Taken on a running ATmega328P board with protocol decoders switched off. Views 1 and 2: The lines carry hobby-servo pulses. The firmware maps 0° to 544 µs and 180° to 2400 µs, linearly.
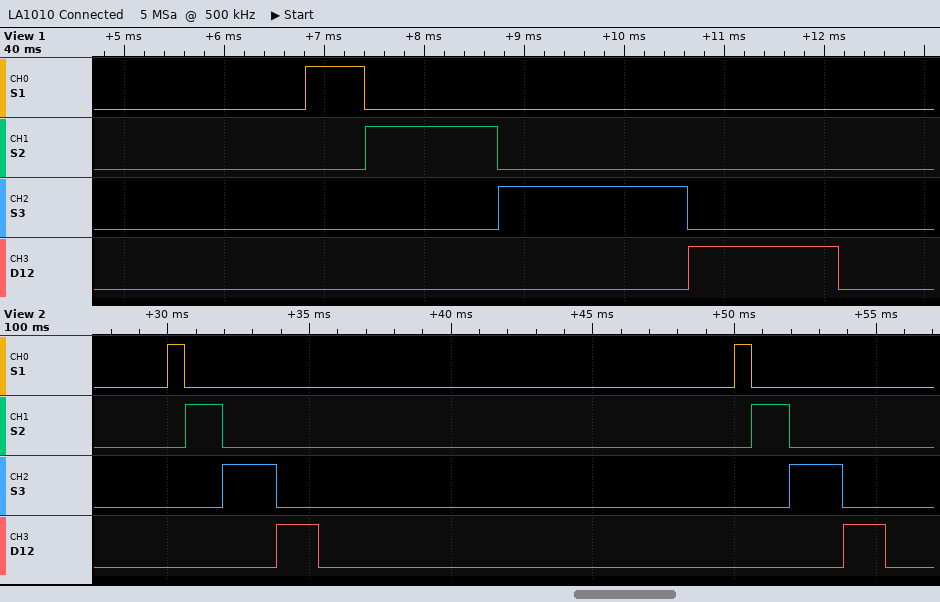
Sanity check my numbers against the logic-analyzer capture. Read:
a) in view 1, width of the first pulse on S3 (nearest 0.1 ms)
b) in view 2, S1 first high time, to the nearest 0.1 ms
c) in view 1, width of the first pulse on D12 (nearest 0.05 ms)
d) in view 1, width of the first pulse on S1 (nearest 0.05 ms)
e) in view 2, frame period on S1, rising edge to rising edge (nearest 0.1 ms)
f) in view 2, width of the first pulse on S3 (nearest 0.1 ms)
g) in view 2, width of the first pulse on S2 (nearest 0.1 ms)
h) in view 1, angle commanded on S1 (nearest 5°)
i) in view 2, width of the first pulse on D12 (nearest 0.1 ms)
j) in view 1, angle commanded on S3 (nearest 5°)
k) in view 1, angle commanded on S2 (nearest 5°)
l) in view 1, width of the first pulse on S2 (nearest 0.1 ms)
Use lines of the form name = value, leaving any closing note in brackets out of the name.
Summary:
in view 1, width of the first pulse on S3 = 1.9 ms
in view 2, S1 first high time, to the nearest 0.1 ms = 0.6 ms
in view 1, width of the first pulse on D12 = 1.50 ms
in view 1, width of the first pulse on S1 = 0.60 ms
in view 2, frame period on S1, rising edge to rising edge = 20.0 ms
in view 2, width of the first pulse on S3 = 1.9 ms
in view 2, width of the first pulse on S2 = 1.3 ms
in view 1, angle commanded on S1 = 5°
in view 2, width of the first pulse on D12 = 1.5 ms
in view 1, angle commanded on S3 = 130°
in view 1, angle commanded on S2 = 75°
in view 1, width of the first pulse on S2 = 1.3 ms
